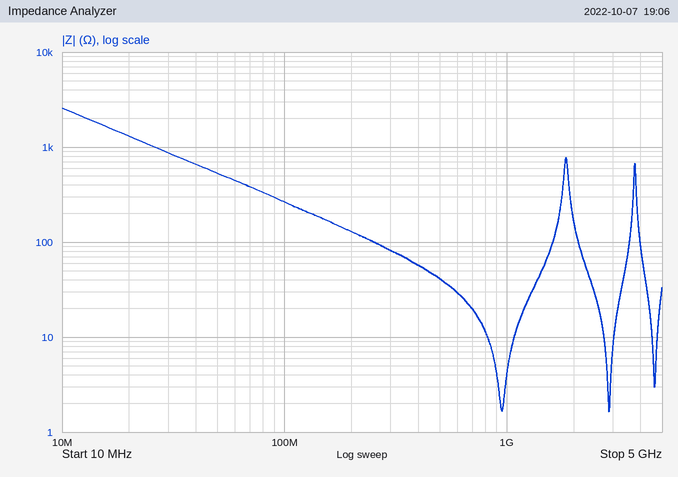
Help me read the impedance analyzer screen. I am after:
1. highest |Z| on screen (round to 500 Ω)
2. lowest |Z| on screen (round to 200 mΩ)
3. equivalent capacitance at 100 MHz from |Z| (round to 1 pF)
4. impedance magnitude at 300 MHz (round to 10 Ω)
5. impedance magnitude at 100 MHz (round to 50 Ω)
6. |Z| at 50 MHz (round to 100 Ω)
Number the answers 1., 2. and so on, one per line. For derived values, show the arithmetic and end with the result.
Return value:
1. 2.5 kΩ
2. 1.6 Ω
3. C = 1/(2π × 100 MHz × 250 Ω) ≈ 6 pF
4. 80 Ω
5. 250 Ω
6. 500 Ω
